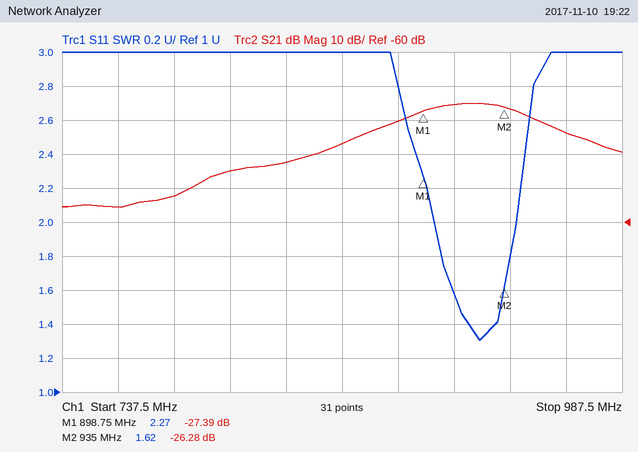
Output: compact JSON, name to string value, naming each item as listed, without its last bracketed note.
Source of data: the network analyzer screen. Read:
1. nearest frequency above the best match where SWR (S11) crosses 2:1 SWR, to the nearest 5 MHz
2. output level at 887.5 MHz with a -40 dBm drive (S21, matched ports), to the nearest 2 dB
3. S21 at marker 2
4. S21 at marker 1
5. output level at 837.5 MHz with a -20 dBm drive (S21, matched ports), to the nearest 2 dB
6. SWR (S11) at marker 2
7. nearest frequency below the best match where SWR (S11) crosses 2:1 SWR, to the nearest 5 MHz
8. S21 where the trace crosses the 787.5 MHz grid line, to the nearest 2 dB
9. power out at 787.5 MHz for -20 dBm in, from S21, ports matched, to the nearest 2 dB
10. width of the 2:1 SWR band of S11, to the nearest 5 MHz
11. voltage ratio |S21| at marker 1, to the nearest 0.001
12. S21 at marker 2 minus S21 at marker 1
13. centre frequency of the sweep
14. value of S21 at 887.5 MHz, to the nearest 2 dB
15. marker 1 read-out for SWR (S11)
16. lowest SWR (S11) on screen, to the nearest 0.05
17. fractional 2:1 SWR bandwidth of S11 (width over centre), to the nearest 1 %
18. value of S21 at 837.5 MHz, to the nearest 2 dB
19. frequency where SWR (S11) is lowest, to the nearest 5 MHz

{"nearest frequency above the best match where SWR (S11) crosses 2:1 SWR, to the nearest 5 MHz": "940 MHz", "output level at 887.5 MHz with a -40 dBm drive (S21, matched ports), to the nearest 2 dB": "-70 dBm", "S21 at marker 2": "-26.28 dB", "S21 at marker 1": "-27.39 dB", "output level at 837.5 MHz with a -20 dBm drive (S21, matched ports), to the nearest 2 dB": "-62 dBm", "SWR (S11) at marker 2": "1.62", "nearest frequency below the best match where SWR (S11) crosses 2:1 SWR, to the nearest 5 MHz": "905 MHz", "S21 where the trace crosses the 787.5 MHz grid line, to the nearest 2 dB": "-52 dB", "power out at 787.5 MHz for -20 dBm in, from S21, ports matched, to the nearest 2 dB": "-72 dBm", "width of the 2:1 SWR band of S11, to the nearest 5 MHz": "35 MHz", "voltage ratio |S21| at marker 1, to the nearest 0.001": "0.043", "S21 at marker 2 minus S21 at marker 1": "1.11 dB", "centre frequency of the sweep": "862.5 MHz", "value of S21 at 887.5 MHz, to the nearest 2 dB": "-30 dB", "marker 1 read-out for SWR": "2.27", "lowest SWR (S11) on screen, to the nearest 0.05": "1.30", "fractional 2:1 SWR bandwidth of S11 (width over centre), to the nearest 1 %": "4 %", "value of S21 at 837.5 MHz, to the nearest 2 dB": "-42 dB", "frequency where SWR (S11) is lowest, to the nearest 5 MHz": "925 MHz"}
